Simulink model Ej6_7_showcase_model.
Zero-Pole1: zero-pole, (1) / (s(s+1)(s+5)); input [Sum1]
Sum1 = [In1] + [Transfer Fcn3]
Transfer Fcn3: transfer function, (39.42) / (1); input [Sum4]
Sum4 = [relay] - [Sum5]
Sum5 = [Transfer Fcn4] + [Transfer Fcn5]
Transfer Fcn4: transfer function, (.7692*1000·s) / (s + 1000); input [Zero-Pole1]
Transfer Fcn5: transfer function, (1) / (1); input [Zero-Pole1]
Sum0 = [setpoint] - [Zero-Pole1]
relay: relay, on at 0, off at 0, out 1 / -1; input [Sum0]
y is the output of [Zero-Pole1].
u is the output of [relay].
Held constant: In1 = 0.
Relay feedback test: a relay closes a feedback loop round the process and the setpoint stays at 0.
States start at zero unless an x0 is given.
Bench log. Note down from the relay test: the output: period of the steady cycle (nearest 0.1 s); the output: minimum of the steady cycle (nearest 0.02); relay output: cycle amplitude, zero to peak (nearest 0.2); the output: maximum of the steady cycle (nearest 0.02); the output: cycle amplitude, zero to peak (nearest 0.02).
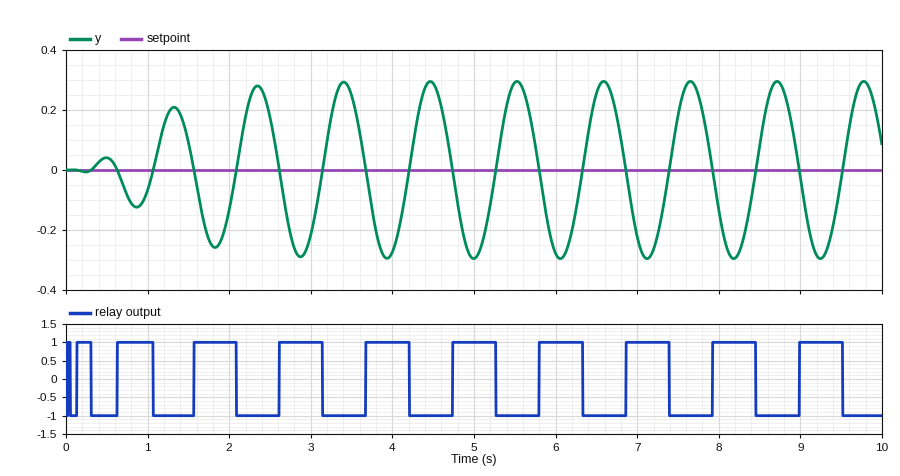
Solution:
1.1 s
-0.30
1.0
0.30
0.30
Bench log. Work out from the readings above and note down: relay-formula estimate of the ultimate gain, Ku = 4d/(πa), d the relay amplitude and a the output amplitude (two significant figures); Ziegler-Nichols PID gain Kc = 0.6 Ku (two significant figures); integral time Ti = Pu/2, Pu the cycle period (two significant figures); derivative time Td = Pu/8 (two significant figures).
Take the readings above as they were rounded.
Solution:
4.2
2.5
0.55 s
0.14 s
